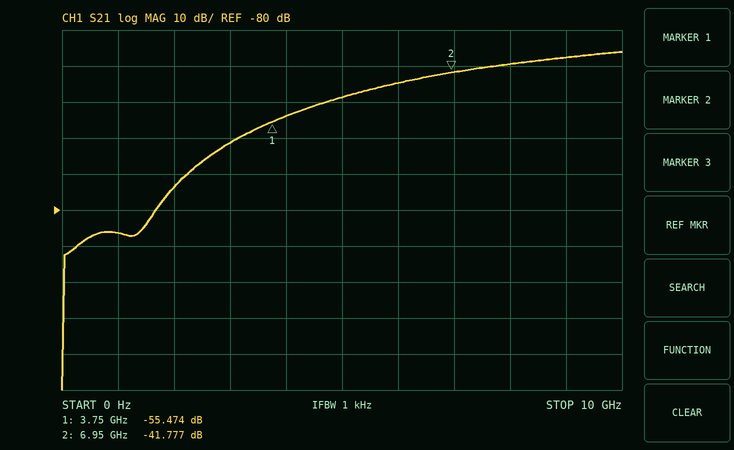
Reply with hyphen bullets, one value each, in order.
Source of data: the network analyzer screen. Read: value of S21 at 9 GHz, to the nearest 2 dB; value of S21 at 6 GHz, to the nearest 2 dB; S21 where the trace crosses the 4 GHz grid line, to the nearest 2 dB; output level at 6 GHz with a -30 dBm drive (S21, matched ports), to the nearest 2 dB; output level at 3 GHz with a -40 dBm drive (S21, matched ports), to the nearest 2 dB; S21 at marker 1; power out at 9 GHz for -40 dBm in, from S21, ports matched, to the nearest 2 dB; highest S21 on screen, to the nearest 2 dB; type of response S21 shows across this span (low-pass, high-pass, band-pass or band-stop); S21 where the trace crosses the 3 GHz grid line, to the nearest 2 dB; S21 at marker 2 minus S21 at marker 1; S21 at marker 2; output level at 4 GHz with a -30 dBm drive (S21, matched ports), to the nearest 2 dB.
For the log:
- -38 dB
- -44 dB
- -54 dB
- -74 dBm
- -102 dBm
- -55.474 dB
- -78 dBm
- -36 dB
- high-pass
- -62 dB
- 13.697 dB
- -41.777 dB
- -84 dBm
